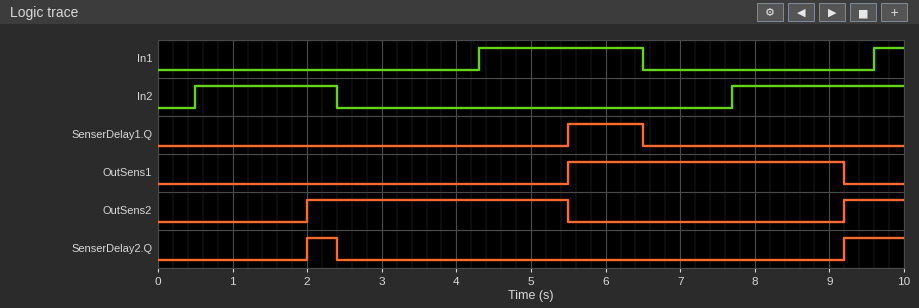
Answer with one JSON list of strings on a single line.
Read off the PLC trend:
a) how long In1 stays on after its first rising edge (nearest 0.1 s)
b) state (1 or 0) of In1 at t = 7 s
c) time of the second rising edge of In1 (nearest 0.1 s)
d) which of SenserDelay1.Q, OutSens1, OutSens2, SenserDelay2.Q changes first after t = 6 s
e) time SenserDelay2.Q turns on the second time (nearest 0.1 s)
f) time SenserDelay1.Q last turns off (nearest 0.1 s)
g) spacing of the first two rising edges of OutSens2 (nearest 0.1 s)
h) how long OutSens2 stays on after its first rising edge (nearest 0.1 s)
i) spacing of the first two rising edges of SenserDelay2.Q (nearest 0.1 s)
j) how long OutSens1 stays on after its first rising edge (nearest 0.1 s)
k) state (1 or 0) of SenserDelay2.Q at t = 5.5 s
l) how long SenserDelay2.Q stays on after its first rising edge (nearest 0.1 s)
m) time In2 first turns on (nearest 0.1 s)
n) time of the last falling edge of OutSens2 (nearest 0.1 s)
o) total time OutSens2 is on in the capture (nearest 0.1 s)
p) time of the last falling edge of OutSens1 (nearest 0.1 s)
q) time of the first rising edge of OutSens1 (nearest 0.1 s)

["2.2 s", "0", "9.6 s", "SenserDelay1.Q", "9.2 s", "6.5 s", "7.2 s", "3.5 s", "7.2 s", "3.7 s", "0", "0.4 s", "0.5 s", "5.5 s", "4.3 s", "9.2 s", "5.5 s"]
